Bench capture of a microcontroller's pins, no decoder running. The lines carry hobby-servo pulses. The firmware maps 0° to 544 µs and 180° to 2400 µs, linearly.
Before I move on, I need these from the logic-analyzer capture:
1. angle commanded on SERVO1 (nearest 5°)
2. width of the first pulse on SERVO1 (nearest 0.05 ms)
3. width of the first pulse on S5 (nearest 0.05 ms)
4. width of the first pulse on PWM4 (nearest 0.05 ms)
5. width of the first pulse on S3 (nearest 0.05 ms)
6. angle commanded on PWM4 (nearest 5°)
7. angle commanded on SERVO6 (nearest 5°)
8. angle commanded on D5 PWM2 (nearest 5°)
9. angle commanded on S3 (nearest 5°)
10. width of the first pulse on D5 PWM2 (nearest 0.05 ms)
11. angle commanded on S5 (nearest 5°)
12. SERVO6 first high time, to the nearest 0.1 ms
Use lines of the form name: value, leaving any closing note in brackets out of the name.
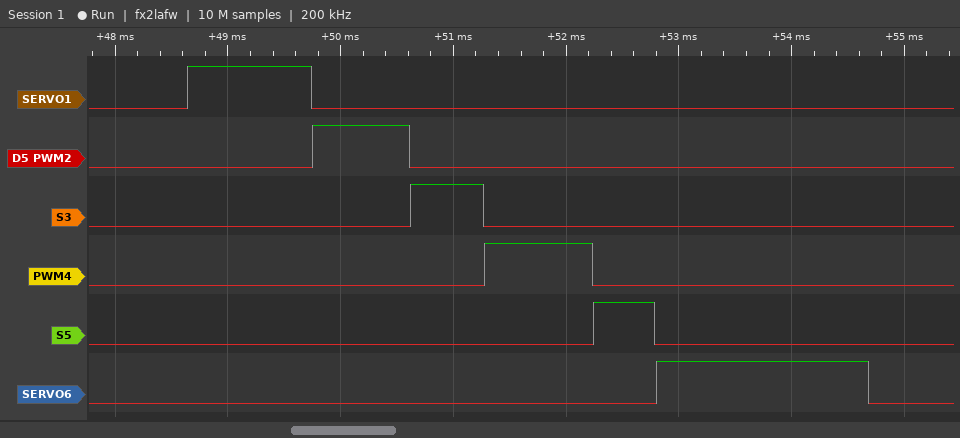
angle commanded on SERVO1: 55°
width of the first pulse on SERVO1: 1.10 ms
width of the first pulse on S5: 0.55 ms
width of the first pulse on PWM4: 0.95 ms
width of the first pulse on S3: 0.65 ms
angle commanded on PWM4: 40°
angle commanded on SERVO6: 130°
angle commanded on D5 PWM2: 30°
angle commanded on S3: 10°
width of the first pulse on D5 PWM2: 0.85 ms
angle commanded on S5: 0°
SERVO6 first high time, to the nearest 0.1 ms: 1.9 ms
